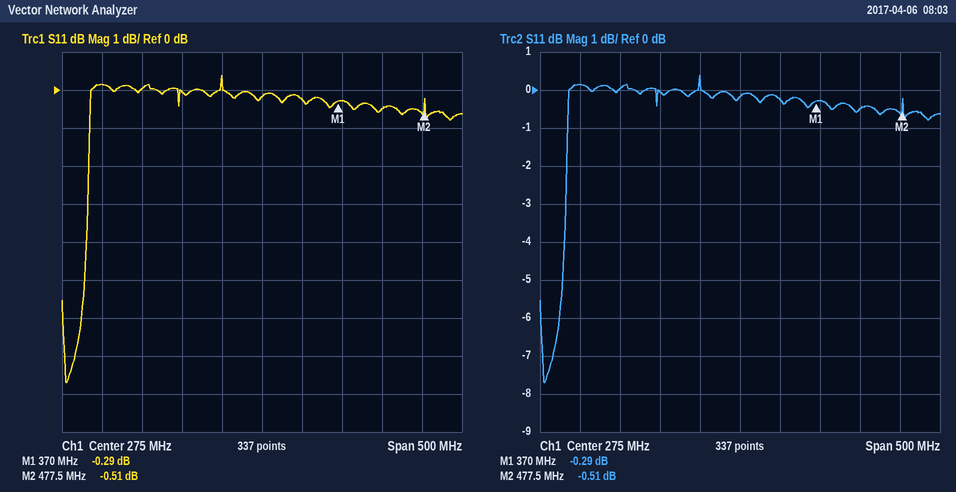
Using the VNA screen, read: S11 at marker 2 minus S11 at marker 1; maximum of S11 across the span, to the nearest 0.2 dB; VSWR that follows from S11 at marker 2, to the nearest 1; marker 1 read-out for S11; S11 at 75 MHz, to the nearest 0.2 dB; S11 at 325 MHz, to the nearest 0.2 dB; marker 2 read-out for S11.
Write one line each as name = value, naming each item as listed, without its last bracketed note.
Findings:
S11 at marker 2 minus S11 at marker 1 = -0.22 dB
maximum of S11 across the span, to the nearest 0.2 dB = 0.4 dB
VSWR that follows from S11 at marker 2, to the nearest 1 = 34
marker 1 read-out for S11 = -0.29 dB
S11 at 75 MHz, to the nearest 0.2 dB = 0.2 dB
S11 at 325 MHz, to the nearest 0.2 dB = -0.2 dB
marker 2 read-out for S11 = -0.51 dB
